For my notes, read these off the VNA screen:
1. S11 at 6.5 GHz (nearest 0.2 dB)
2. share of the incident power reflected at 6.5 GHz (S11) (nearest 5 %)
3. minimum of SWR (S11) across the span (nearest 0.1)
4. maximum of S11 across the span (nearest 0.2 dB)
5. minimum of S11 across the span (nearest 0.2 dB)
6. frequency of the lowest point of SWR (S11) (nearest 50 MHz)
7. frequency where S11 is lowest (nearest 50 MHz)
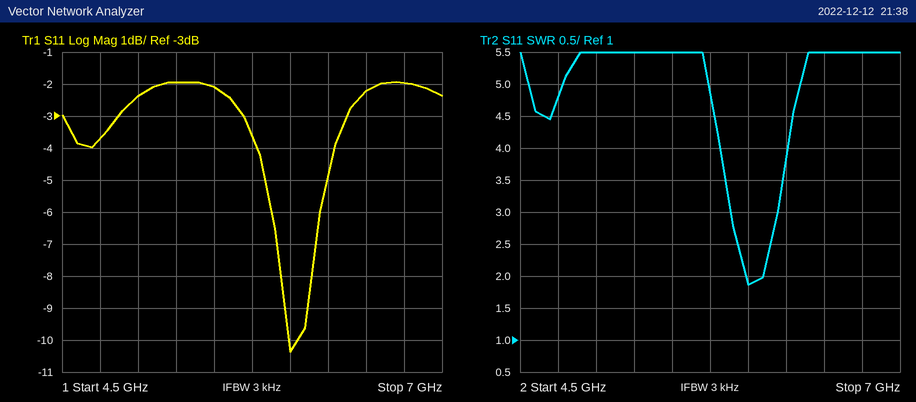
-2.2 dB
60 %
1.9
-2.0 dB
-10.4 dB
6.00 GHz
6.00 GHz
